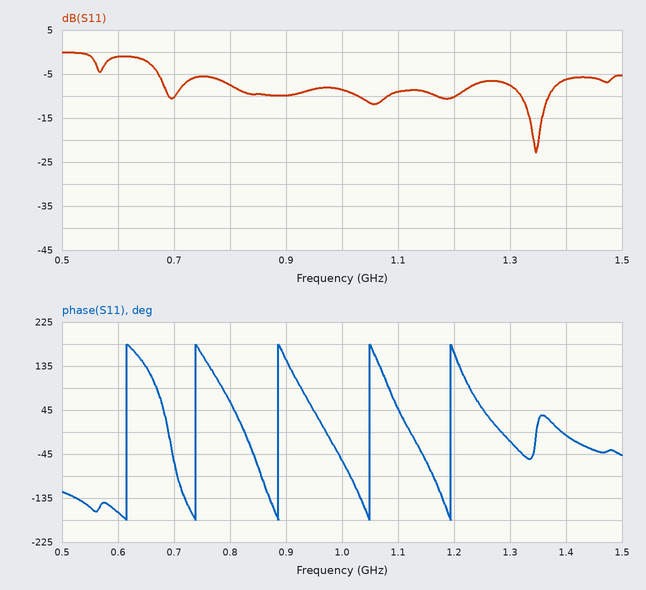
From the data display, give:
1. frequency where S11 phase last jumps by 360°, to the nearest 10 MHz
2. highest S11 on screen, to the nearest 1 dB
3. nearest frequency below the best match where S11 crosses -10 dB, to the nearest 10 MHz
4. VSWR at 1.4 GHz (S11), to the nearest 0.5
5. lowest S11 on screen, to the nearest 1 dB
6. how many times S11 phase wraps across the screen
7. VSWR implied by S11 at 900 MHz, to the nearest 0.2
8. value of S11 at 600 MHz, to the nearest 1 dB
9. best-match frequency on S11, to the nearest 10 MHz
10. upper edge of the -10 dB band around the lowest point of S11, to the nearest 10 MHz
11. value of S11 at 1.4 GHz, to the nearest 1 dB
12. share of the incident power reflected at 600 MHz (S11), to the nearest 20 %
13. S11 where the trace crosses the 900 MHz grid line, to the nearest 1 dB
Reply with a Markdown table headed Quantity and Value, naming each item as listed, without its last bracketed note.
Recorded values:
| Quantity | Value |
|---|---|
| frequency where S11 phase last jumps by 360°, to the nearest 10 MHz | 1.19 GHz |
| highest S11 on screen, to the nearest 1 dB | 0 dB |
| nearest frequency below the best match where S11 crosses -10 dB, to the nearest 10 MHz | 1.32 GHz |
| VSWR at 1.4 GHz (S11), to the nearest 0.5 | 3.0 |
| lowest S11 on screen, to the nearest 1 dB | -23 dB |
| how many times S11 phase wraps across the screen | 5 |
| VSWR implied by S11 at 900 MHz, to the nearest 0.2 | 2.0 |
| value of S11 at 600 MHz, to the nearest 1 dB | -1 dB |
| best-match frequency on S11, to the nearest 10 MHz | 1.35 GHz |
| upper edge of the -10 dB band around the lowest point of S11, to the nearest 10 MHz | 1.37 GHz |
| value of S11 at 1.4 GHz, to the nearest 1 dB | -6 dB |
| share of the incident power reflected at 600 MHz (S11), to the nearest 20 % | 80 % |
| S11 where the trace crosses the 900 MHz grid line, to the nearest 1 dB | -10 dB |
